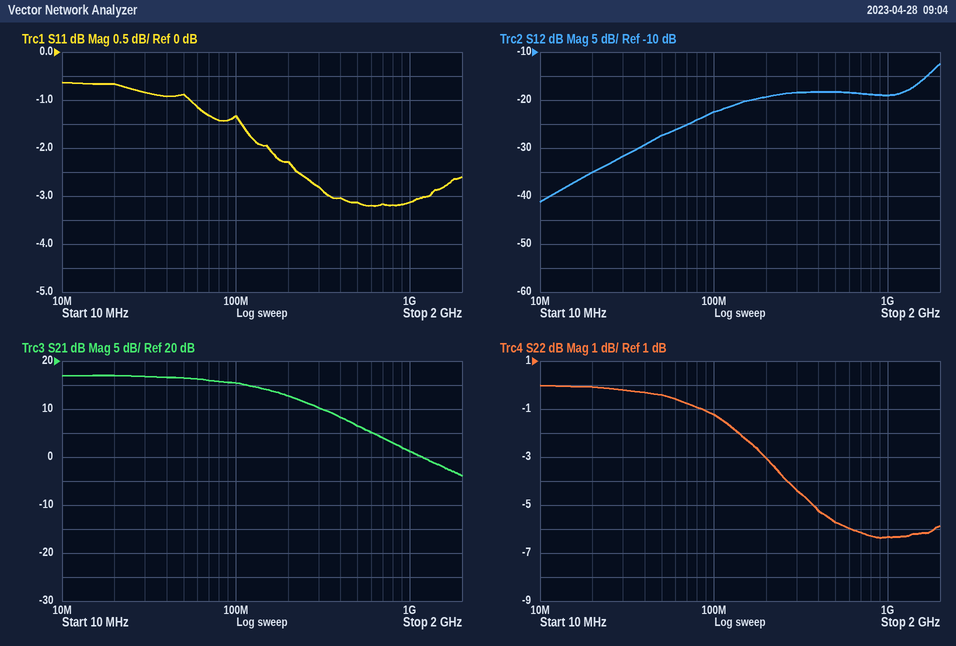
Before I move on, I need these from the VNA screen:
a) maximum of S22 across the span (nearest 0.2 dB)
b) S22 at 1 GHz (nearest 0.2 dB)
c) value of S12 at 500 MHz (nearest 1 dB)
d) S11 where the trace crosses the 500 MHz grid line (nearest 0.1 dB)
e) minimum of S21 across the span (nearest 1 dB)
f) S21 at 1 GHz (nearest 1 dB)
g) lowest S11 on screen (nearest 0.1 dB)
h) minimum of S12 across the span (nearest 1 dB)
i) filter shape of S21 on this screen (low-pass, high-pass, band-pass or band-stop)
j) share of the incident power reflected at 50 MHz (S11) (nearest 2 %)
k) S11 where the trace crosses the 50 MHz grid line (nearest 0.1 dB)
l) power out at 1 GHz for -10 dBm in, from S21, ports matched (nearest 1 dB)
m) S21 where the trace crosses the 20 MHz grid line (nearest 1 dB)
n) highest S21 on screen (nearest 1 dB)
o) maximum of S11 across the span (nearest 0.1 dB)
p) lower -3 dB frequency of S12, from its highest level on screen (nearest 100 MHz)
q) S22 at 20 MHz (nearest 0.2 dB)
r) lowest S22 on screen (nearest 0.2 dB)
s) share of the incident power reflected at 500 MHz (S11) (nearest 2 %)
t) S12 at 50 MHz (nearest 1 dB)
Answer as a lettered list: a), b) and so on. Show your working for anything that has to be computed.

a) 0.0 dB
b) -6.4 dB
c) -18 dB
d) -3.1 dB
e) -4 dB
f) 1 dB
g) -3.2 dB
h) -41 dB
i) low-pass
j) 10^(-0.9/10) ≈ 81.3 %, so 82 % to the nearest 2 %
k) -0.9 dB
l) -10 dBm + (1 dB) = -9 dBm
m) 17 dB
n) 17 dB
o) -0.6 dB
p) 1.6 GHz
q) 0.0 dB
r) -6.4 dB
s) 10^(-3.1/10) ≈ 49.0 %, so 48 % to the nearest 2 %
t) -27 dB
